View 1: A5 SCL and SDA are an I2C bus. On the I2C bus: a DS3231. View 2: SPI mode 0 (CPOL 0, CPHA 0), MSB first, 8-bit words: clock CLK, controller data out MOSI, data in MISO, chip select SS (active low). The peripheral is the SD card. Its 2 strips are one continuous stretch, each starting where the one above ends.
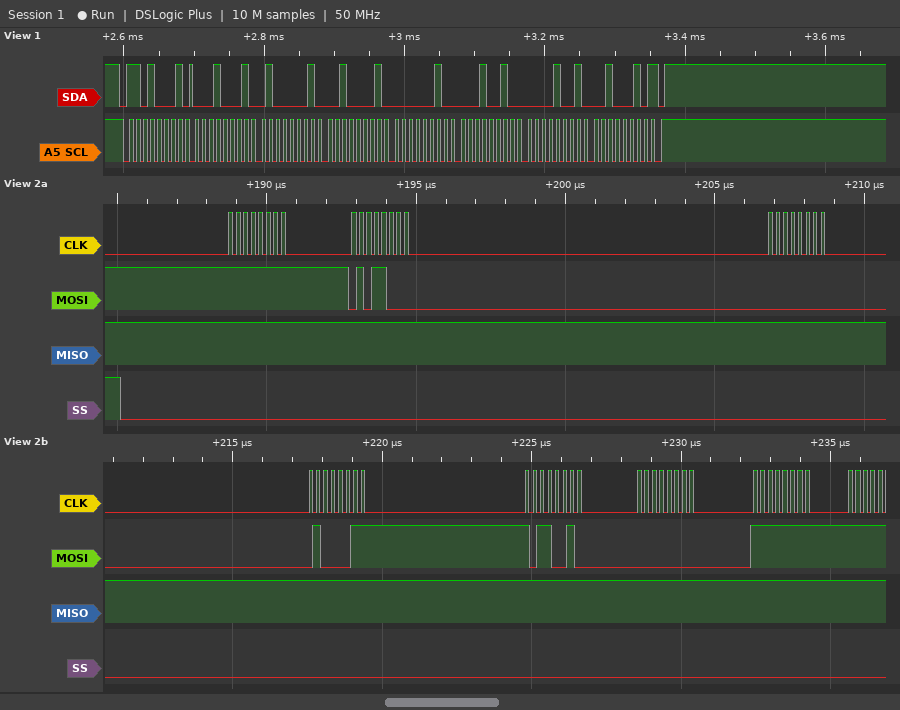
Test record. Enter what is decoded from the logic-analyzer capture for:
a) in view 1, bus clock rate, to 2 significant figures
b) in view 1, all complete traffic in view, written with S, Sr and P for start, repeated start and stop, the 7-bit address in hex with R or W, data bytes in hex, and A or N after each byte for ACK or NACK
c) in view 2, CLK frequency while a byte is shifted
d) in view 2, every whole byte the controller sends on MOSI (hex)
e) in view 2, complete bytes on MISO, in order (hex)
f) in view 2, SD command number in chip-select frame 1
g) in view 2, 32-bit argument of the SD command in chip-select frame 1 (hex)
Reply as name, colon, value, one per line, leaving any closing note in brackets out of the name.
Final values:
in view 1, bus clock rate, to 2 significant figures: 100 kHz
in view 1, all complete traffic in view, written with S, Sr and P for start, repeated start and stop, the 7-bit address in hex with R or W, data bytes in hex, and A or N after each byte for ACK or NACK: S 68R A 11 A 41 A 21 A 02 A 12 A 09 A 22 N P
in view 2, CLK frequency while a byte is shifted: 4 MHz
in view 2, every whole byte the controller sends on MOSI: 0xFF 0x58 0x00 0x43 0xB2 0x00 0xFF
in view 2, complete bytes on MISO, in order: 0xFF 0xFF 0xFF 0xFF 0xFF 0xFF 0xFF
in view 2, SD command number in chip-select frame 1: CMD24
in view 2, 32-bit argument of the SD command in chip-select frame 1: 0x0043B200
